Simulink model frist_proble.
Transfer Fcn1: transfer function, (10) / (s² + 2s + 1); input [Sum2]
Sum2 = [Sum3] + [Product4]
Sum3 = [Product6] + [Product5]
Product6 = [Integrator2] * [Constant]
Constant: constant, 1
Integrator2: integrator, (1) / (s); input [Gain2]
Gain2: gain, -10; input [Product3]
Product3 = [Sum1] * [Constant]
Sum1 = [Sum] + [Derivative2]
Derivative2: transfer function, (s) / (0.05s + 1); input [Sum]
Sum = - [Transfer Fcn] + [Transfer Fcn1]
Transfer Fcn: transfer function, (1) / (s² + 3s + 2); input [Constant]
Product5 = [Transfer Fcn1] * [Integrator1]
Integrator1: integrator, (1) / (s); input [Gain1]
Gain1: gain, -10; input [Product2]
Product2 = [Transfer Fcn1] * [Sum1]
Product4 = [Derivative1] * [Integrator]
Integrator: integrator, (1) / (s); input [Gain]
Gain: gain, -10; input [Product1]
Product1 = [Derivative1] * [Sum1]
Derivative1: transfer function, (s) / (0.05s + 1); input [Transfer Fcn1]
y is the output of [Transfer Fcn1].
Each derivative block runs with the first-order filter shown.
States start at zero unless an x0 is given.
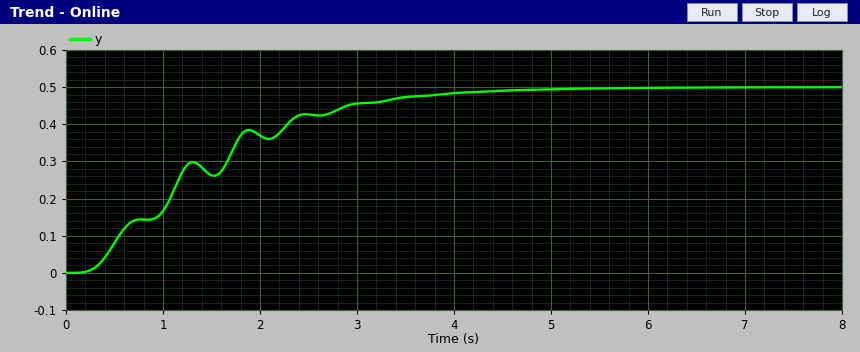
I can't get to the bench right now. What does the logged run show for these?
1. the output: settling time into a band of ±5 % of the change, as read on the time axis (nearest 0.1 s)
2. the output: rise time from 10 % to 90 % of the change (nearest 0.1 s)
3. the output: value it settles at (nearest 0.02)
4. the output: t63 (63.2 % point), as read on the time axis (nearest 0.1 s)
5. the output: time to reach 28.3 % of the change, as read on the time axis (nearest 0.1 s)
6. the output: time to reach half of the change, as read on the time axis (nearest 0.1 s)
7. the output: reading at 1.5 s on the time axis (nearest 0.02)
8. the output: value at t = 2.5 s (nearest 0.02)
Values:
3.6 s
2.5 s
0.50
1.7 s
0.7 s
1.2 s
0.26
0.42
